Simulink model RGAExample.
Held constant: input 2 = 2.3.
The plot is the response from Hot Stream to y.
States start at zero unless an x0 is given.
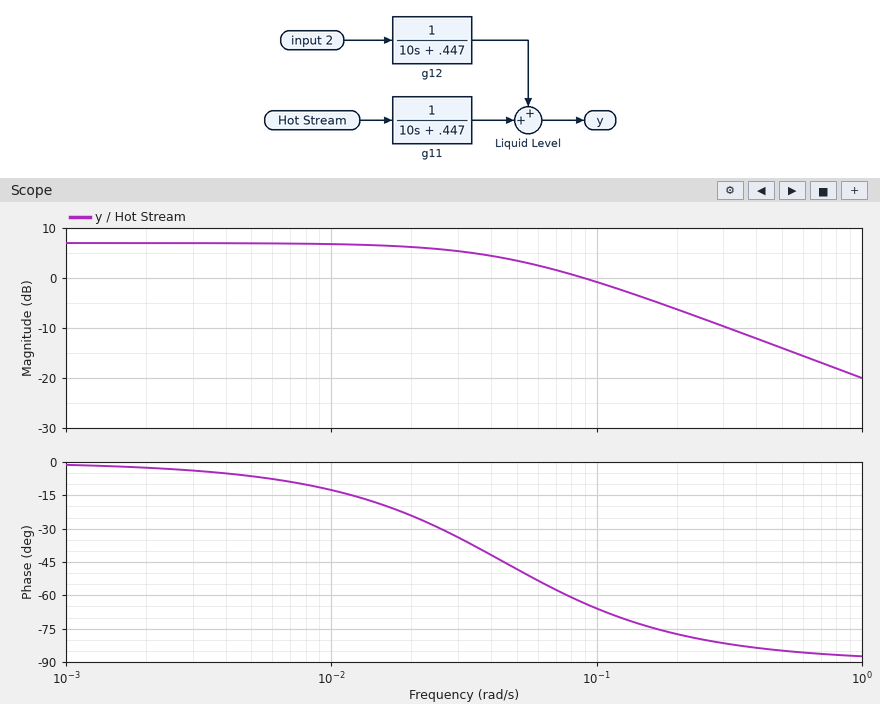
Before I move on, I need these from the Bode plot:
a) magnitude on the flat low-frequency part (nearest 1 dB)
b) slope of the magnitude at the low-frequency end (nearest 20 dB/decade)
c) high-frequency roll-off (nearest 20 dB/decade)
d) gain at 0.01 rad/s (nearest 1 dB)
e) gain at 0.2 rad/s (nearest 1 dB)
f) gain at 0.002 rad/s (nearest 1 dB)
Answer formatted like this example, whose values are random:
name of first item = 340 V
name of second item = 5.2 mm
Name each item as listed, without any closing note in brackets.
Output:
magnitude on the flat low-frequency part = 7 dB
slope of the magnitude at the low-frequency end = 0 dB/decade
high-frequency roll-off = -20 dB/decade
gain at 0.01 rad/s = 7 dB
gain at 0.2 rad/s = -6 dB
gain at 0.002 rad/s = 7 dB
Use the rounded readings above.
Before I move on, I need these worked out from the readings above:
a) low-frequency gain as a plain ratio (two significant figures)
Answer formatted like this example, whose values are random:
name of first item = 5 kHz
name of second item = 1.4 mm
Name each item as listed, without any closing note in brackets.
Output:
low-frequency gain as a plain ratio = 2.2
